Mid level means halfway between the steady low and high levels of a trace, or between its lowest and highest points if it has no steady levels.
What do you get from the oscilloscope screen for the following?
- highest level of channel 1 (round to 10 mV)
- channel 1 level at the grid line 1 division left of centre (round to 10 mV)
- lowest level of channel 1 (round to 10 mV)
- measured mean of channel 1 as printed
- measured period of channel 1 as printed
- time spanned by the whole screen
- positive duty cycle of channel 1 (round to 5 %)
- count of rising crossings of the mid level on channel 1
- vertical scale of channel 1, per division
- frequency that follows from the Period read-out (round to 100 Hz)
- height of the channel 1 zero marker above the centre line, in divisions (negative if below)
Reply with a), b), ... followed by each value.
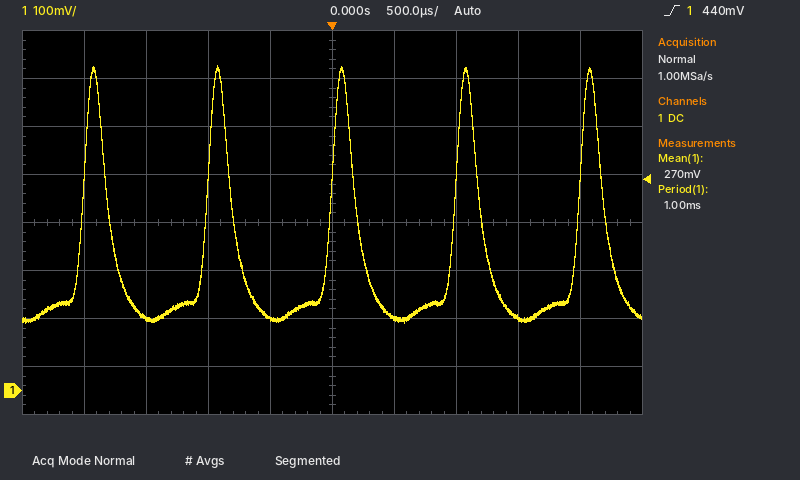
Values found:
a) 680 mV
b) 150 mV
c) 140 mV
d) 270 mV
e) 1.00 ms
f) 5 ms
g) 20 %
h) 5
i) 100 mV
j) 1.0 kHz
k) -3.5 div
